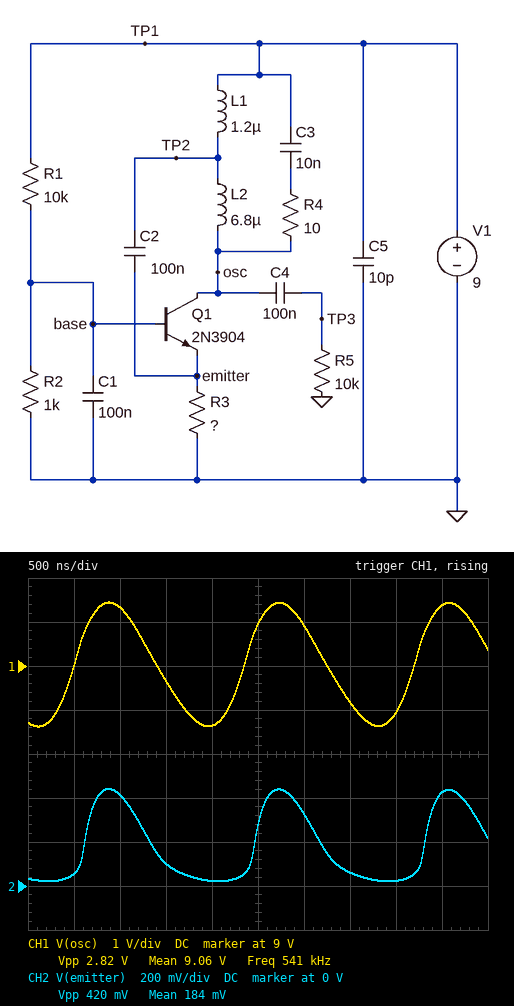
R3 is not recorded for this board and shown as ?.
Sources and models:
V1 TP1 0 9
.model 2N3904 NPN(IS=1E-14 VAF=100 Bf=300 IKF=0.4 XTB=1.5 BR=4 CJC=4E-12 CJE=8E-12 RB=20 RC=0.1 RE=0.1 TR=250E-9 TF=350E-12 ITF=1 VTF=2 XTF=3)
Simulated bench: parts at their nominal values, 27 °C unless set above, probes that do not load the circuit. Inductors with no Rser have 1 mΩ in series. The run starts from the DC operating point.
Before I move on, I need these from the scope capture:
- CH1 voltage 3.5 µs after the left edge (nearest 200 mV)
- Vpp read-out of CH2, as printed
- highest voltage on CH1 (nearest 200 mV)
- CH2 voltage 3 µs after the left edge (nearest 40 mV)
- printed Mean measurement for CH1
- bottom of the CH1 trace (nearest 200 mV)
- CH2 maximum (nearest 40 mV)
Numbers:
8.2 V
420 mV
10.4 V
320 mV
9.06 V
7.6 V
440 mV
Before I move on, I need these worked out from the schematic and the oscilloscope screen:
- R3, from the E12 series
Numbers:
12 Ω
